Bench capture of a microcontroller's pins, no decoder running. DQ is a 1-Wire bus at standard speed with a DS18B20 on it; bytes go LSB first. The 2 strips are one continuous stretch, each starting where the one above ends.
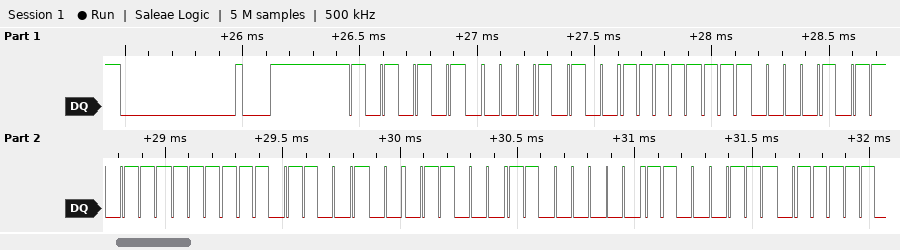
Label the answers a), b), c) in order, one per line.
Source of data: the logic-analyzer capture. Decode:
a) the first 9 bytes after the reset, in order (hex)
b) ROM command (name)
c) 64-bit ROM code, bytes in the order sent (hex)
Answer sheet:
a) 55 28 FF D0 FE 9B 18 03 E3
b) Match ROM
c) 28 FF D0 FE 9B 18 03 E3
